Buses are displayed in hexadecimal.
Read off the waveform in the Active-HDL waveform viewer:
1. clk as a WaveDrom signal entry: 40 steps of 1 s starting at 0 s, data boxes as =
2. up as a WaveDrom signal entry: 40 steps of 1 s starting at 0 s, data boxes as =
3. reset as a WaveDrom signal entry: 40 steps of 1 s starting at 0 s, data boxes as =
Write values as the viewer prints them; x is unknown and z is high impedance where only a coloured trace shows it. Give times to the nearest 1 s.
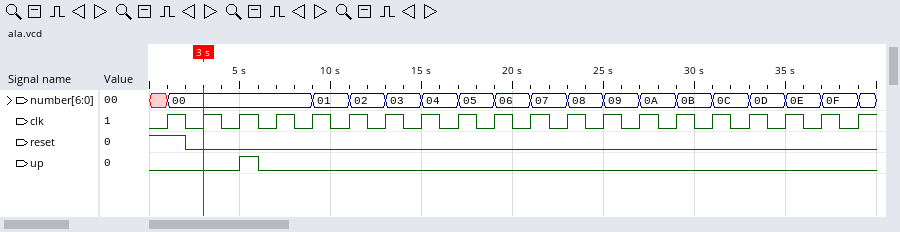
{name: 'clk', wave: '0101010101010101010101010101010101010101'}
{name: 'up', wave: '0....10.................................'}
{name: 'reset', wave: '1.0.....................................'}
